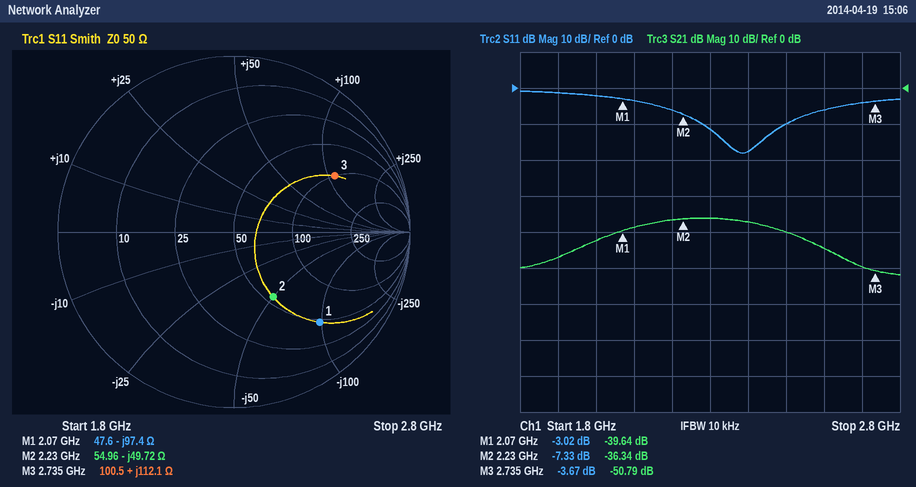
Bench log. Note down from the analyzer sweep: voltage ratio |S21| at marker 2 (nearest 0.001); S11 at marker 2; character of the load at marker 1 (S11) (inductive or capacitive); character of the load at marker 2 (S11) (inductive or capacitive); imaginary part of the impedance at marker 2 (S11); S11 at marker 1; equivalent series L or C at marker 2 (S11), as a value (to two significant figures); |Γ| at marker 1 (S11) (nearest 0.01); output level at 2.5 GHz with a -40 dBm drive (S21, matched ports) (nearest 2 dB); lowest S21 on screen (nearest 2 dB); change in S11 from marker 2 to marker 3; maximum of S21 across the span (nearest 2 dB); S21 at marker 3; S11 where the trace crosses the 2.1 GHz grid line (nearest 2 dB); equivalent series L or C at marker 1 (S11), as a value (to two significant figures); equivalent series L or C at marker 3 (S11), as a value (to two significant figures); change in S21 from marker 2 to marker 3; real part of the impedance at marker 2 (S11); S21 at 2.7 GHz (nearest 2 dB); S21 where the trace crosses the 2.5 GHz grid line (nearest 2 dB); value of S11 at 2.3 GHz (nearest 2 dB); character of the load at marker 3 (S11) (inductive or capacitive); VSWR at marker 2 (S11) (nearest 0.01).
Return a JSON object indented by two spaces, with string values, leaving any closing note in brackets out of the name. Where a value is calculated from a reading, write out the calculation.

{
  "voltage ratio |S21| at marker 2": "10^(-36.34/20) ≈ 0.015",
  "S11 at marker 2": "-7.33 dB",
  "character of the load at marker 1 (S11)": "capacitive",
  "character of the load at marker 2 (S11)": "capacitive",
  "imaginary part of the impedance at marker 2": "-49.72 Ω",
  "S11 at marker 1": "-3.02 dB",
  "equivalent series L or C at marker 2 (S11), as a value": "C = 1/(2π × 2.23 GHz × 49.72 Ω) ≈ 1.4 pF",
  "|Γ| at marker 1 (S11)": "0.71",
  "output level at 2.5 GHz with a -40 dBm drive (S21, matched ports)": "-40 dBm + (-40 dB) = -80 dBm",
  "lowest S21 on screen": "-52 dB",
  "change in S11 from marker 2 to marker 3": "-3.67 − (-7.33) = 3.66 dB",
  "maximum of S21 across the span": "-36 dB",
  "S21 at marker 3": "-50.79 dB",
  "S11 where the trace crosses the 2.1 GHz grid line": "-4 dB",
  "equivalent series L or C at marker 1 (S11), as a value": "C = 1/(2π × 2.07 GHz × 97.4 Ω) ≈ 789 fF, so 790 fF to two significant figures",
  "equivalent series L or C at marker 3 (S11), as a value": "L = 112.1 Ω/(2π × 2.735 GHz) ≈ 6.5 nH",
  "change in S21 from marker 2 to marker 3": "-50.79 − (-36.34) = -14.45 dB",
  "real part of the impedance at marker 2": "54.96 Ω",
  "S21 at 2.7 GHz": "-50 dB",
  "S21 where the trace crosses the 2.5 GHz grid line": "-40 dB",
  "value of S11 at 2.3 GHz": "-12 dB",
  "character of the load at marker 3 (S11)": "inductive",
  "VSWR at marker 2 (S11)": "(1 + 0.4300)/(1 − 0.4300) ≈ 2.51"
}
